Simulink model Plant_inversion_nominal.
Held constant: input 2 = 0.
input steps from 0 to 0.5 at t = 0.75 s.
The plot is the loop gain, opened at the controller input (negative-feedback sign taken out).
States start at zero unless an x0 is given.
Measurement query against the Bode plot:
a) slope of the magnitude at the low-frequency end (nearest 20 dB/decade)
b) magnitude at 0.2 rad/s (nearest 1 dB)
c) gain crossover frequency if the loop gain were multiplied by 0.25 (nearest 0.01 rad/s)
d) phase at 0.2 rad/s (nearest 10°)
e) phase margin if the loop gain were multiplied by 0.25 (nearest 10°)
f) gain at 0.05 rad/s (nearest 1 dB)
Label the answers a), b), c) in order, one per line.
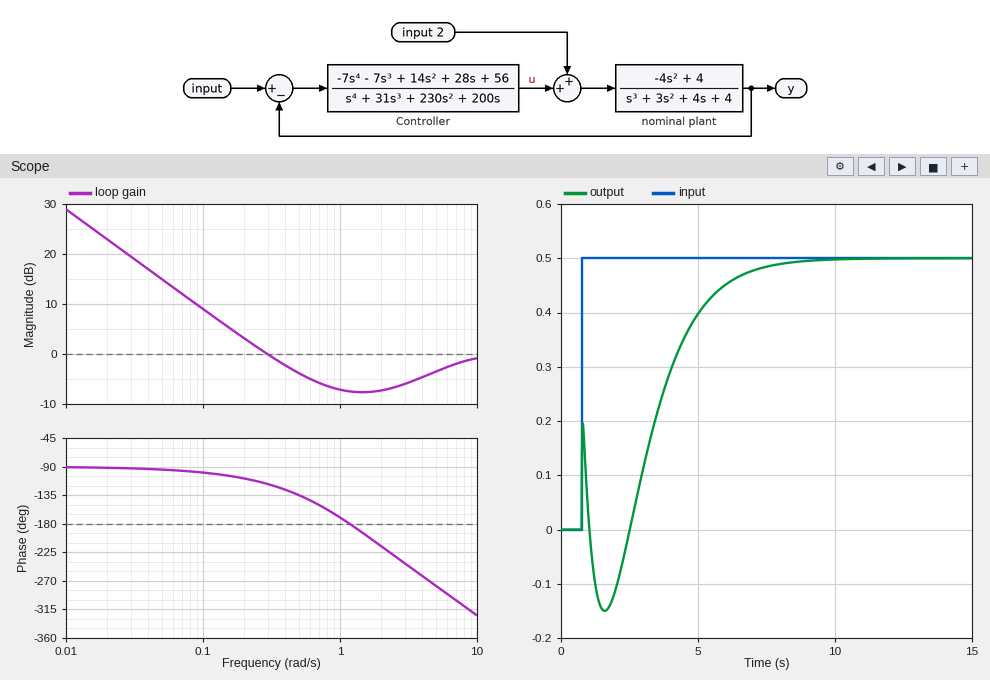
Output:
a) -20 dB/decade
b) 3 dB
c) 0.07 rad/s
d) -110°
e) 80°
f) 15 dB
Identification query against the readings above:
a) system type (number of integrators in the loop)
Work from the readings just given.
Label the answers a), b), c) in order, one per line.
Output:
a) 1
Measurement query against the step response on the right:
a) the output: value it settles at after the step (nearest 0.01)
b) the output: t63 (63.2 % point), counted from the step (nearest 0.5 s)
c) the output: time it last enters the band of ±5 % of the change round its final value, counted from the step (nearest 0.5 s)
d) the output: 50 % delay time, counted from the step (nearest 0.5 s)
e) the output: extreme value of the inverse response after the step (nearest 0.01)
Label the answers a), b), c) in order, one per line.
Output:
a) 0.50
b) 3.5 s
c) 6.0 s
d) 3.0 s
e) -0.15
